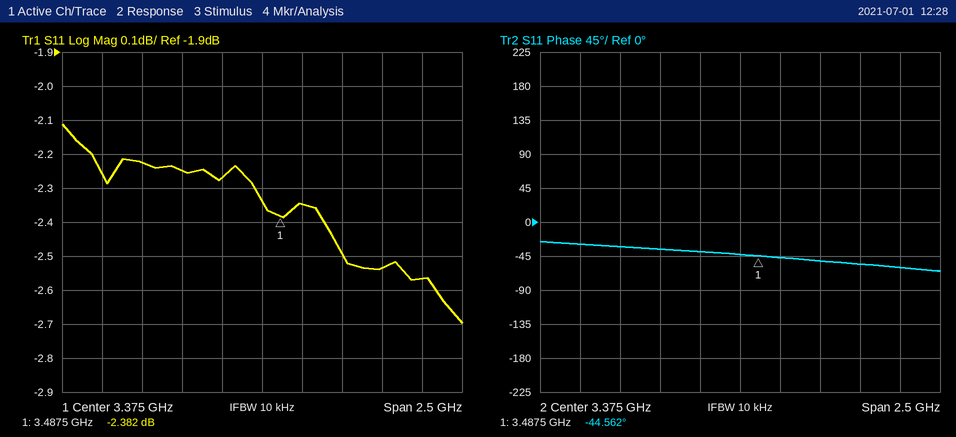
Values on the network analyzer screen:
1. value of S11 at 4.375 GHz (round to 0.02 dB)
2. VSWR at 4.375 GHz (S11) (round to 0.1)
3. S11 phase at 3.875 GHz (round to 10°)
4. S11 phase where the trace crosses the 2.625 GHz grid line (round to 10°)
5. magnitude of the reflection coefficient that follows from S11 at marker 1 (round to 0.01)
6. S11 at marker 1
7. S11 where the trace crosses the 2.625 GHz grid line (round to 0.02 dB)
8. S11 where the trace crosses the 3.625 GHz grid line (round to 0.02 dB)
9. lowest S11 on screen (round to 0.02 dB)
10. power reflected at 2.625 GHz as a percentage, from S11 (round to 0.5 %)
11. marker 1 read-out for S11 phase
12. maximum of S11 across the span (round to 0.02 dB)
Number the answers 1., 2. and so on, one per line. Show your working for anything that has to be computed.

1. -2.56 dB
2. |Γ| = 10^(-2.56/20) = 0.7447; VSWR = (1 + 0.7447)/(1 − 0.7447) ≈ 6.8
3. -50°
4. -30°
5. 10^(-2.382/20) ≈ 0.76
6. -2.382 dB
7. -2.22 dB
8. -2.34 dB
9. -2.70 dB
10. 10^(-2.22/10) ≈ 60.0 %
11. -44.562°
12. -2.12 dB
